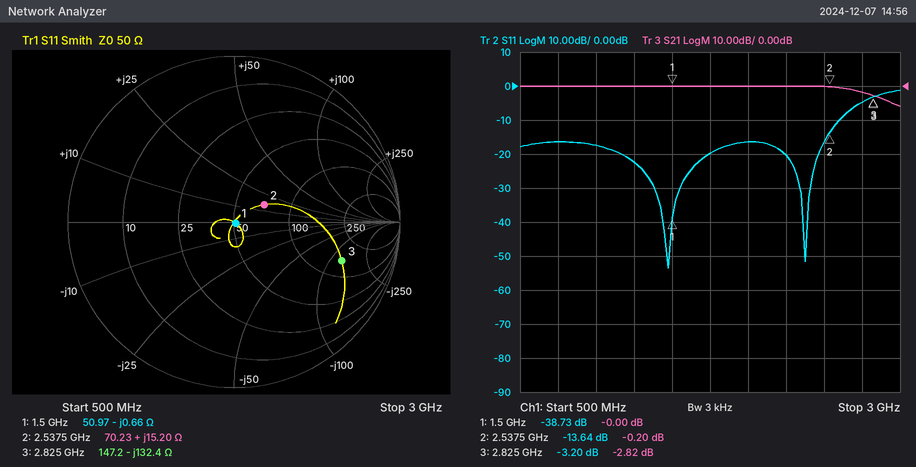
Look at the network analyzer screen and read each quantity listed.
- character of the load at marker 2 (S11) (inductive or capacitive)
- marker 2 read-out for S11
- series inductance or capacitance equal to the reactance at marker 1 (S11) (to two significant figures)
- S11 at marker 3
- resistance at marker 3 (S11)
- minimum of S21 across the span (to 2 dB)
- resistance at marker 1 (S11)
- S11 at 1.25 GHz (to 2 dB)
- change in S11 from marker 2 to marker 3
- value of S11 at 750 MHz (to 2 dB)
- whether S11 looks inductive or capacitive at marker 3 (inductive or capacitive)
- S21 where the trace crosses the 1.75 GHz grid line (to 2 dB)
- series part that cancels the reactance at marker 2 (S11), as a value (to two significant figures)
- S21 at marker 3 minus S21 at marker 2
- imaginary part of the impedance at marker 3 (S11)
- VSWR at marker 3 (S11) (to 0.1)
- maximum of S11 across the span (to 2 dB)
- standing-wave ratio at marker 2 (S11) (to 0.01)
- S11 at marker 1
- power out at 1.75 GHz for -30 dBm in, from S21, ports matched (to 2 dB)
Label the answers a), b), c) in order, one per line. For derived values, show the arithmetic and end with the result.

a) inductive
b) -13.64 dB
c) C = 1/(2π × 1.5 GHz × 0.66 Ω) ≈ 161 pF, so 160 pF to two significant figures
d) -3.20 dB
e) 147.2 Ω
f) -6 dB
g) 50.97 Ω
h) -22 dB
i) -3.2 − (-13.64) = 10.44 dB
j) -16 dB
k) capacitive
l) 0 dB
m) C = 1/(2π × 2.5375 GHz × 15.2 Ω) ≈ 4.1 pF
n) -2.82 − (-0.2) = -2.62 dB
o) -132.4 Ω
p) 5.5
q) -2 dB
r) 1.53
s) -38.73 dB
t) -30 dBm + (0 dB) = -30 dBm
